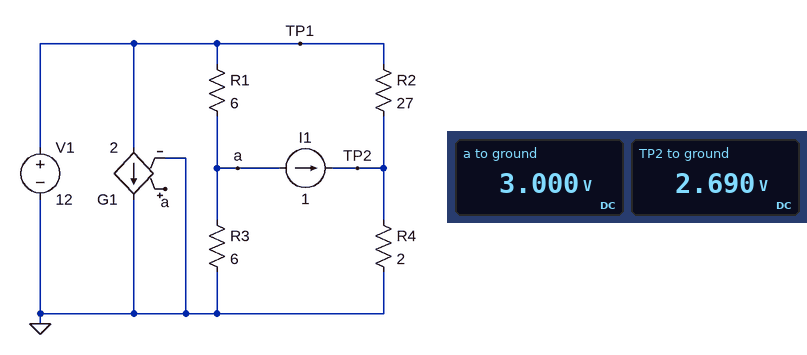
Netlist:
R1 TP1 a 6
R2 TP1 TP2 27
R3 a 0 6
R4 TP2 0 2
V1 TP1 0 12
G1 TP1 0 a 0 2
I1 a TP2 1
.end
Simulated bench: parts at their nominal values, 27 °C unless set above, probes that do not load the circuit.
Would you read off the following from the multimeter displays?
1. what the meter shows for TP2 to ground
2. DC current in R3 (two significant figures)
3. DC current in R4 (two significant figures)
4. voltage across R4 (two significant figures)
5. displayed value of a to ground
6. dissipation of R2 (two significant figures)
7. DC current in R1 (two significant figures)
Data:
2.690 V
500 mA
1.3 A
2.7 V
3.000 V
3.2 W
1.5 A
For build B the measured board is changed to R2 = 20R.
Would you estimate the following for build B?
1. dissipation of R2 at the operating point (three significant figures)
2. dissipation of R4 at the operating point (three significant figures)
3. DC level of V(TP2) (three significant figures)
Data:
4.13 W
4.23 W
2.91 V
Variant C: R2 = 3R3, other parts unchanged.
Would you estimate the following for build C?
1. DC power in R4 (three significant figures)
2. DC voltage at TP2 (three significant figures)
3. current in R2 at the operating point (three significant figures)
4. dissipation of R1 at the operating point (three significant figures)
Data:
16.7 W
5.77 V
1.89 A
13.5 W
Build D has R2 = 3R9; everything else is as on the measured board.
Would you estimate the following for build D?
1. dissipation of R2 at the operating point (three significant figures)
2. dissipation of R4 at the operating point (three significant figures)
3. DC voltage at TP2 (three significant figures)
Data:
11.2 W
14.5 W
5.39 V
